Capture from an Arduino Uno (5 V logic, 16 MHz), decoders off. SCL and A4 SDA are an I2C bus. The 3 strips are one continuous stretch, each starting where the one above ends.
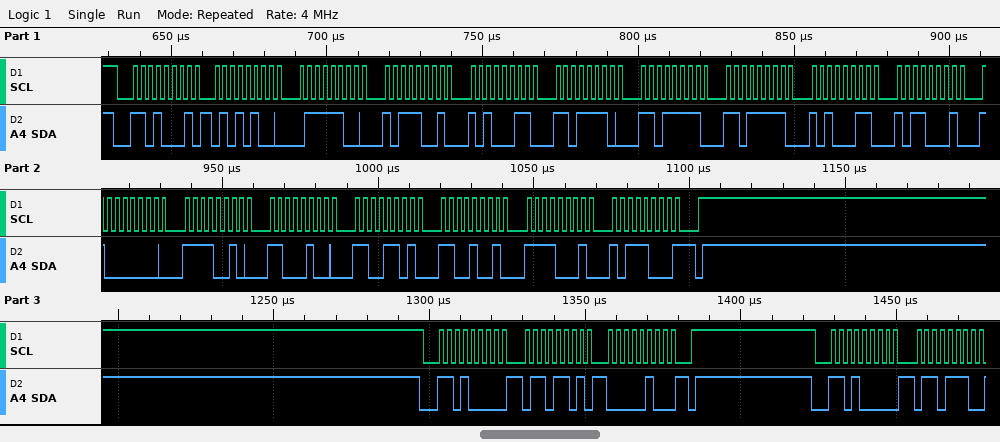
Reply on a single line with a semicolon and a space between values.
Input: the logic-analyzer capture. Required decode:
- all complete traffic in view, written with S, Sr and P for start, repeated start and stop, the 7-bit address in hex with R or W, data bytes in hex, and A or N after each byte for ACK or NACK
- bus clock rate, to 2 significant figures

S 68R A 54 A 7C A B9 A A3 A DE A DF A DF A A3 A B1 A 80 A F2 A C4 A CD A C9 A F1 A B8 N P S 68W A 6D A 04 A P S 68W A 6E A; 400 kHz
